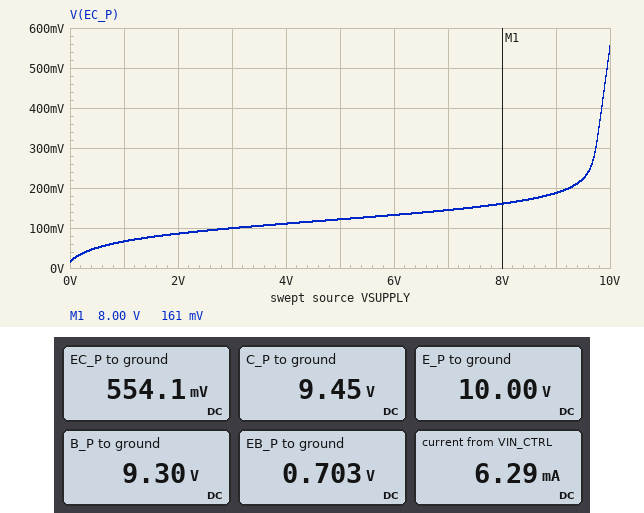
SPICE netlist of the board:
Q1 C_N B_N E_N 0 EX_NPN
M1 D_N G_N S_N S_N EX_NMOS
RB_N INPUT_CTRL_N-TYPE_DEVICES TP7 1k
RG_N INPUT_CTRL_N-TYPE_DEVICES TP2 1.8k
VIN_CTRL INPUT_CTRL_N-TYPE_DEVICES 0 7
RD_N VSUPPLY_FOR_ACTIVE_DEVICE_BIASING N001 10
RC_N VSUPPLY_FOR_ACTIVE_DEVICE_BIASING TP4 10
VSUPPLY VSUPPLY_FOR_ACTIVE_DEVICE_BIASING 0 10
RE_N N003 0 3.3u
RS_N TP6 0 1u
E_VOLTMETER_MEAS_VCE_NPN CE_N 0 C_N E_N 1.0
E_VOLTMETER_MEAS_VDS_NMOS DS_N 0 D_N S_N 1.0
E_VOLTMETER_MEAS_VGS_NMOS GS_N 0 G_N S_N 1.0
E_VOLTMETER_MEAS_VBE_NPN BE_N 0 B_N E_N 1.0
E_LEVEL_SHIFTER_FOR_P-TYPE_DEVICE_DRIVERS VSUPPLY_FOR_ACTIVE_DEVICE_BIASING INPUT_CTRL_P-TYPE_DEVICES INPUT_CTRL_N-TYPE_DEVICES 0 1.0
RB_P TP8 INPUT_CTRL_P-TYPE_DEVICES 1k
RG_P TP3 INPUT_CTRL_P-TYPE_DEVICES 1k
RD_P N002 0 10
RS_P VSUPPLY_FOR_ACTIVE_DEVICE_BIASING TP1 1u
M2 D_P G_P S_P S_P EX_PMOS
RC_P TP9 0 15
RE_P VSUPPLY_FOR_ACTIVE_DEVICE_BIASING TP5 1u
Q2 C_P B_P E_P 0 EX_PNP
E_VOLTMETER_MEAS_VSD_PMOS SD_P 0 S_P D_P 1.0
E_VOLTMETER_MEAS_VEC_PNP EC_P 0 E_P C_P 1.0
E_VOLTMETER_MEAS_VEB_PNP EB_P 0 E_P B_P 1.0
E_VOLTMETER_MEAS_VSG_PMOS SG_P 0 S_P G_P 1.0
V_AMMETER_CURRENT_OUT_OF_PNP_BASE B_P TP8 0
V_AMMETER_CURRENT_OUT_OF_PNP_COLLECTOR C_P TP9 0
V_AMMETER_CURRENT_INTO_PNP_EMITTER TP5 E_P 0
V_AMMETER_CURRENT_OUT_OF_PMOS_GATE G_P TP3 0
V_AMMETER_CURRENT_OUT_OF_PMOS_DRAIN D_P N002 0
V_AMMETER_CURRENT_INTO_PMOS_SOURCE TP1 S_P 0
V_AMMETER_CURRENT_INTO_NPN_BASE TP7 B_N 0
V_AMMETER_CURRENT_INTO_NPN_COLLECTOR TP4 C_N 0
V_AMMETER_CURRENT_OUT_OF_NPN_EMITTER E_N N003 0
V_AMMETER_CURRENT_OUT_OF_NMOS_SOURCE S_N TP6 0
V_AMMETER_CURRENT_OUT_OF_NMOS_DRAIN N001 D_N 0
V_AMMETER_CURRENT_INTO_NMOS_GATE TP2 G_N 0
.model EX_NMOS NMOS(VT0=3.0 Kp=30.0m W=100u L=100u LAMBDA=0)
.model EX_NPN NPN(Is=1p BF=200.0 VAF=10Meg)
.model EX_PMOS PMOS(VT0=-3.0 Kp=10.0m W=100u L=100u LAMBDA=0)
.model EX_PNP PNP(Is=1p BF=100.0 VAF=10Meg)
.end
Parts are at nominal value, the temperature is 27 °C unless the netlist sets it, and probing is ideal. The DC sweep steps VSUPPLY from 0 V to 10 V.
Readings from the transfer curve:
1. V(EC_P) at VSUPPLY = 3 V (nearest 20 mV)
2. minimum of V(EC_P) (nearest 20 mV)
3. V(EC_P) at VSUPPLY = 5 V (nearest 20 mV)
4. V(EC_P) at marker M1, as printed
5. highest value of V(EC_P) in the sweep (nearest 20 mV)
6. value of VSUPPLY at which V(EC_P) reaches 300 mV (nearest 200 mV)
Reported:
100 mV
20 mV
120 mV
161 mV
560 mV
9.8 V
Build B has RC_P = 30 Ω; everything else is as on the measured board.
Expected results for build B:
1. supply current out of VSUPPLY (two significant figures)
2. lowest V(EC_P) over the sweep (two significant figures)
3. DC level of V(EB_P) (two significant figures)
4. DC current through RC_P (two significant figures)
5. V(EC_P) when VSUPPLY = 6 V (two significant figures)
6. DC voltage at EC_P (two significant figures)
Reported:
1.6 A
17 mV
690 mV
330 mA
100 mV
120 mV
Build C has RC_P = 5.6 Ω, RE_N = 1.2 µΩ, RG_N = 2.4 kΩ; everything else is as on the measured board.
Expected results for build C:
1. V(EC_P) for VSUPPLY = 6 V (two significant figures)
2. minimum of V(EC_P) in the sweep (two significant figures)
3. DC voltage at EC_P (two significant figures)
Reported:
2.5 V
13 mV
6.5 V
